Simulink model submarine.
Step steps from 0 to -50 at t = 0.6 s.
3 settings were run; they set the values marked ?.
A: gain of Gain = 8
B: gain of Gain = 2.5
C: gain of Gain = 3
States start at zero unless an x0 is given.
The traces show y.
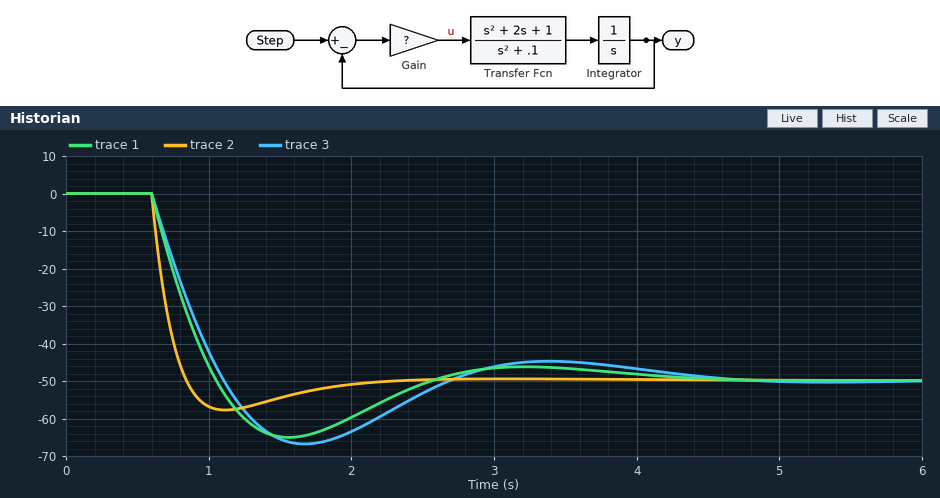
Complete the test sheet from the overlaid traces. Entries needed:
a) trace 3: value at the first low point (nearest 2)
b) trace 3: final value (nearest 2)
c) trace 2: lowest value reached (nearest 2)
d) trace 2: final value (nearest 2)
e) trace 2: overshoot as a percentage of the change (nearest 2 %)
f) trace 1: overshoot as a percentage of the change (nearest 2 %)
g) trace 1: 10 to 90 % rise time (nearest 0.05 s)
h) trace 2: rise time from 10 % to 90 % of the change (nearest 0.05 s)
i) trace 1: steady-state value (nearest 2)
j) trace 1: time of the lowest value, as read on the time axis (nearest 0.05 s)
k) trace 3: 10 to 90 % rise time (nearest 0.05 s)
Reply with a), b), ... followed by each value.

a) -66
b) -50
c) -58
d) -50
e) 16 %
f) 30 %
g) 0.35 s
h) 0.20 s
i) -50
j) 1.55 s
k) 0.40 s
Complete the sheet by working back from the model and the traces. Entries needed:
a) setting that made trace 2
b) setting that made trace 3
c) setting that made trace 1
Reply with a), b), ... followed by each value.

a) A
b) B
c) C
